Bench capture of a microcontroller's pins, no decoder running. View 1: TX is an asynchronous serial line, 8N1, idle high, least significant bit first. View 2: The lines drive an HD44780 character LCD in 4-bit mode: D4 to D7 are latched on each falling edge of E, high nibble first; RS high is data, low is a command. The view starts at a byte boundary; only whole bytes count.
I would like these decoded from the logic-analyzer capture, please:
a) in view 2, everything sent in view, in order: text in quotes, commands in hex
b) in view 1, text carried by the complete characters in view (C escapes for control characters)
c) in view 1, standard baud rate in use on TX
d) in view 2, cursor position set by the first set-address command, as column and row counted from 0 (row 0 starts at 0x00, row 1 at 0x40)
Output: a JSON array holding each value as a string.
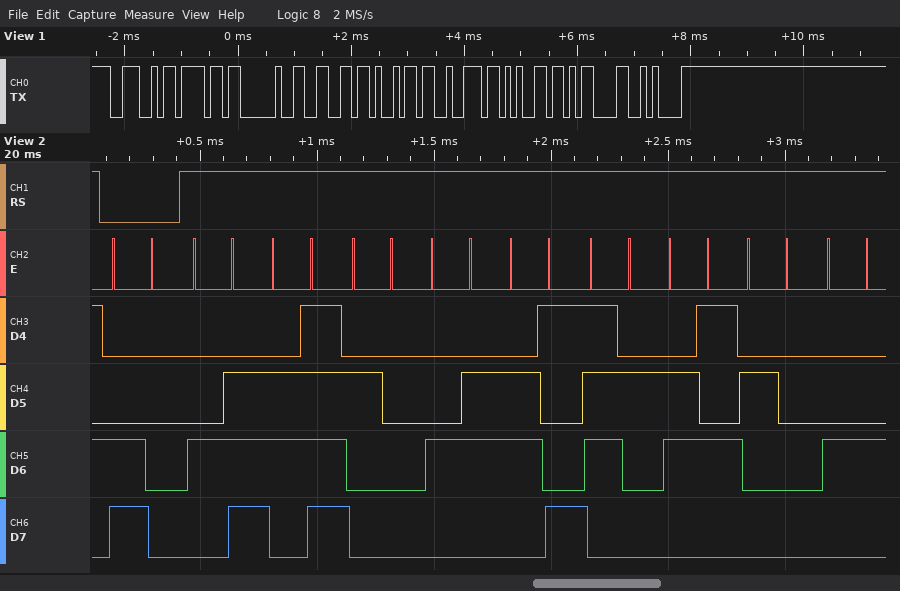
["0xC0 \"No Fire D\"", "\"No fire\\r\\n\"", "9600 baud", "column 0, row 1"]
